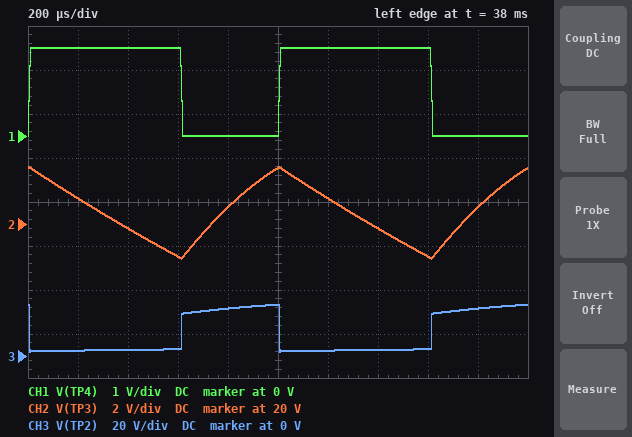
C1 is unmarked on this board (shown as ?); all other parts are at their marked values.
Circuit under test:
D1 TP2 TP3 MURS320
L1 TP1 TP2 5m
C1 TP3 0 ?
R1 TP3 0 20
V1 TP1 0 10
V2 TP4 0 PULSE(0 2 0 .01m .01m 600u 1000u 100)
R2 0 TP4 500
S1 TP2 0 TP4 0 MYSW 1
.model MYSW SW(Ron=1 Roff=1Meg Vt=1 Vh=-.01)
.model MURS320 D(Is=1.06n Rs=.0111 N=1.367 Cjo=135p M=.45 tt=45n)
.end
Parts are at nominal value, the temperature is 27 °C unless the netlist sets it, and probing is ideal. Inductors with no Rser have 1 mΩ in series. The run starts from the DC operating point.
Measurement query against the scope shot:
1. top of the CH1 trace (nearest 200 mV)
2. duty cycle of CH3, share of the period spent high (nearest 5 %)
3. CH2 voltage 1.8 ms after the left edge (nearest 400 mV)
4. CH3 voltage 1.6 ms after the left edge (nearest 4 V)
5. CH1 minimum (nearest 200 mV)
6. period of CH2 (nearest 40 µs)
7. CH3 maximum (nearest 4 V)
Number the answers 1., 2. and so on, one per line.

1. 2.0 V
2. 40 %
3. 20.8 V
4. 4 V
5. 0 V
6. 1.00 ms
7. 24 V
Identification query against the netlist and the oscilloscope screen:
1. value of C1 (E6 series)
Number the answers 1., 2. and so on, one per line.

1. 150 µF
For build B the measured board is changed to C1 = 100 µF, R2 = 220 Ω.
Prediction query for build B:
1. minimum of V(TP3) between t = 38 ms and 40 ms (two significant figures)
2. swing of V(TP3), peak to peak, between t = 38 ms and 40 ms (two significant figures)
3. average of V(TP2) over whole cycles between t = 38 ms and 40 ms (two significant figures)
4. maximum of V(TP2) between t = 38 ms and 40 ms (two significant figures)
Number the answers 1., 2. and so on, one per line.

1. 17 V
2. 6.2 V
3. 10 V
4. 24 V
